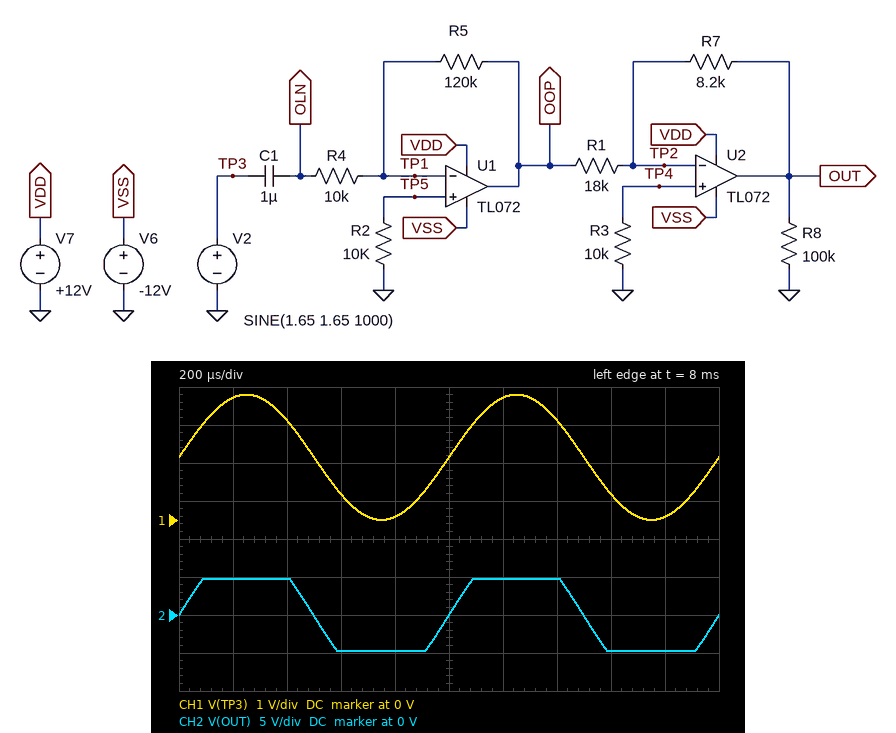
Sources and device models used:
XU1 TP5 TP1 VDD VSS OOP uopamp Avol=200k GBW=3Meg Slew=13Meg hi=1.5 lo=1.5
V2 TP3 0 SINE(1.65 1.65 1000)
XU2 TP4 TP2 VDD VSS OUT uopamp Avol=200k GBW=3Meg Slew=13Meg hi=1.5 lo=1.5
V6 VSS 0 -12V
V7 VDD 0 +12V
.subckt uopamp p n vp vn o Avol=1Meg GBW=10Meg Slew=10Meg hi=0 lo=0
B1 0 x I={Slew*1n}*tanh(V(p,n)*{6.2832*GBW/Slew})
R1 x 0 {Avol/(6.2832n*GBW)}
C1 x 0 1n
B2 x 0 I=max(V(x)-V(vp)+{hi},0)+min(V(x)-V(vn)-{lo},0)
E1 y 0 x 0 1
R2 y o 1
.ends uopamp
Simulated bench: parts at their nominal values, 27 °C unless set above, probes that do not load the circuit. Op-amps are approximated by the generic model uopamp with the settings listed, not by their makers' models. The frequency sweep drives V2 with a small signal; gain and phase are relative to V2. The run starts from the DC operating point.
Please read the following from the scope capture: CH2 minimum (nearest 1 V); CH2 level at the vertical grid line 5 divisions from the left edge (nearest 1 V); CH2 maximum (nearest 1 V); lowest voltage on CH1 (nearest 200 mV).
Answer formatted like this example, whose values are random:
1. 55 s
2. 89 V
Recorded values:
1. -5 V
2. 0 V
3. 5 V
4. 0 V
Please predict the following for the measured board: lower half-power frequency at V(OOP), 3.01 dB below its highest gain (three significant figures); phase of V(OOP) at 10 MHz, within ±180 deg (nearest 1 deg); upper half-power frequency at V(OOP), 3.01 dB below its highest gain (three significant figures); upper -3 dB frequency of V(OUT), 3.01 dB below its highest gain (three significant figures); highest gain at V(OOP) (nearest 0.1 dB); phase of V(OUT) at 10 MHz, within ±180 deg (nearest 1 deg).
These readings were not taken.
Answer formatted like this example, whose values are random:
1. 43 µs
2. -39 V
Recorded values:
1. 15.9 Hz
2. 91 deg
3. 231 kHz
4. 228 kHz
5. 21.6 dB
6. -167 deg
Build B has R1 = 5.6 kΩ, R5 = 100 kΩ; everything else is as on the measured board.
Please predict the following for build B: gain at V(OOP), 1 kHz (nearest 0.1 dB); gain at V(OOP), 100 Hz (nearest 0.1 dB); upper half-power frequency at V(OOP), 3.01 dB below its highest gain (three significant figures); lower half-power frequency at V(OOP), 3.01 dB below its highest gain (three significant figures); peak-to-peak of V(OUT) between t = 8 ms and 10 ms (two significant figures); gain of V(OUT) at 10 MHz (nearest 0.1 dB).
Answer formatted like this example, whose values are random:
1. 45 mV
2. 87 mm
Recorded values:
1. 20.0 dB
2. 19.9 dB
3. 273 kHz
4. 15.9 Hz
5. 21 V
6. -26.3 dB
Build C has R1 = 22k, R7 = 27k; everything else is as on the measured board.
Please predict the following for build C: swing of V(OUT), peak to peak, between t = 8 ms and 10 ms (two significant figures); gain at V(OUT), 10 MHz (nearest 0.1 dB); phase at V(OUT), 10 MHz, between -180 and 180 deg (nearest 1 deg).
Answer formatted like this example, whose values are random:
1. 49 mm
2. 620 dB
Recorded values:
1. 21 V
2. -26.9 dB
3. -171 deg
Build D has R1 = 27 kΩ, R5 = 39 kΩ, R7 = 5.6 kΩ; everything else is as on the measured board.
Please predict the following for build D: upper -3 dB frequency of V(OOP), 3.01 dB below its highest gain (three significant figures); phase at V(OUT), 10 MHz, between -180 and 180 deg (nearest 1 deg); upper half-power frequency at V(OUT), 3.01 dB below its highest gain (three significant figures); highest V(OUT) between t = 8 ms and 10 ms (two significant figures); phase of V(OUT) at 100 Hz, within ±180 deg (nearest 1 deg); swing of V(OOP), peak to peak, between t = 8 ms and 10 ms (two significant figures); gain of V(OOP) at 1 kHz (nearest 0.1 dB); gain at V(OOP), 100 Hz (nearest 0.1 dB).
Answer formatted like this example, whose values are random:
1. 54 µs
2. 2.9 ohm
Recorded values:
1. 612 kHz
2. -163 deg
3. 580 kHz
4. 1.3 V
5. 9 deg
6. 13 V
7. 11.8 dB
8. 11.7 dB
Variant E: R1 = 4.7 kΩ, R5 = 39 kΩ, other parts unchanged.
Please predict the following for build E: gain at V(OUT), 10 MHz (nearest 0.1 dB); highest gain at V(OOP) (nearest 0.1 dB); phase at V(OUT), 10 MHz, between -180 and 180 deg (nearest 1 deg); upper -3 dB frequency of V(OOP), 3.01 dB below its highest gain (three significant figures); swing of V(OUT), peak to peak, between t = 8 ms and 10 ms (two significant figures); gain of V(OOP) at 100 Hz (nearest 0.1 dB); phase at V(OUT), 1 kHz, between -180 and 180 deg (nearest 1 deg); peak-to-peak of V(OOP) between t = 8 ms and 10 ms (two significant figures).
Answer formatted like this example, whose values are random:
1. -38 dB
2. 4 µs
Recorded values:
1. -26.9 dB
2. 11.8 dB
3. -170 deg
4. 612 kHz
5. 21 V
6. 11.7 dB
7. 1 deg
8. 13 V
